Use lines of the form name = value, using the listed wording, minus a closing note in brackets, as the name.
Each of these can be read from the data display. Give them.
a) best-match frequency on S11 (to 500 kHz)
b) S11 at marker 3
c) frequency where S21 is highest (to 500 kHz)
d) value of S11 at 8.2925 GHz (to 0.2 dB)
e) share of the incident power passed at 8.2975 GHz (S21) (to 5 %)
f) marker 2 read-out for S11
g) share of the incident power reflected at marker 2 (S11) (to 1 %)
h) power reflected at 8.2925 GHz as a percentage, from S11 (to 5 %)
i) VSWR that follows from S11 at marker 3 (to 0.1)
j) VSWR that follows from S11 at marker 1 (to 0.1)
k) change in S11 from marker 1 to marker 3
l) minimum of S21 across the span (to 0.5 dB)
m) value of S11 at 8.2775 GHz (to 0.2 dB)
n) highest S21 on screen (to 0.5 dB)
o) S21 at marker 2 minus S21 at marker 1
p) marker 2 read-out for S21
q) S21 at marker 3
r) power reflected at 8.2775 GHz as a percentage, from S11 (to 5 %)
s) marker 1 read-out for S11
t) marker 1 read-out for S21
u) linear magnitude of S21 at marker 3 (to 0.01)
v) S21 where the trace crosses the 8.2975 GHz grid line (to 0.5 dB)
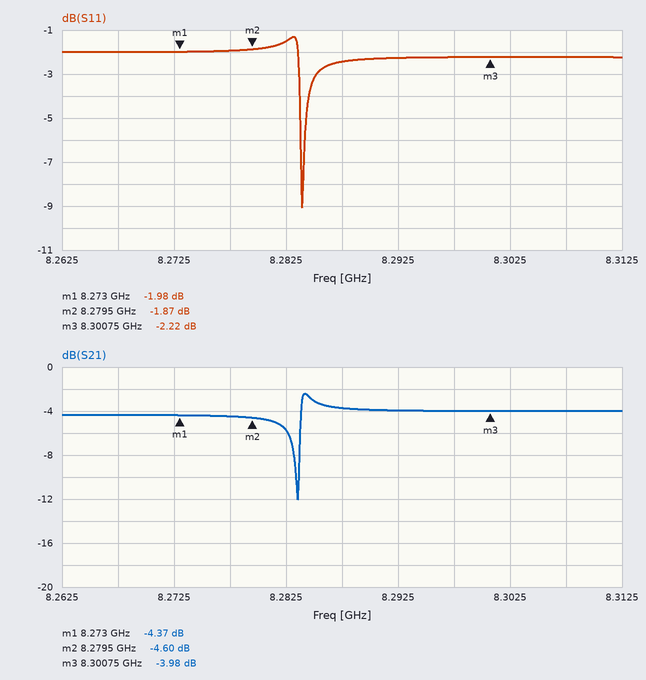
best-match frequency on S11 = 8.2840 GHz
S11 at marker 3 = -2.22 dB
frequency where S21 is highest = 8.2840 GHz
value of S11 at 8.2925 GHz = -2.2 dB
share of the incident power passed at 8.2975 GHz (S21) = 40 %
marker 2 read-out for S11 = -1.87 dB
share of the incident power reflected at marker 2 (S11) = 65 %
power reflected at 8.2925 GHz as a percentage, from S11 = 60 %
VSWR that follows from S11 at marker 3 = 7.9
VSWR that follows from S11 at marker 1 = 8.8
change in S11 from marker 1 to marker 3 = -0.24 dB
minimum of S21 across the span = -12.0 dB
value of S11 at 8.2775 GHz = -2.0 dB
highest S21 on screen = -2.5 dB
S21 at marker 2 minus S21 at marker 1 = -0.23 dB
marker 2 read-out for S21 = -4.60 dB
S21 at marker 3 = -3.98 dB
power reflected at 8.2775 GHz as a percentage, from S11 = 65 %
marker 1 read-out for S11 = -1.98 dB
marker 1 read-out for S21 = -4.37 dB
linear magnitude of S21 at marker 3 = 0.63
S21 where the trace crosses the 8.2975 GHz grid line = -4.0 dB
